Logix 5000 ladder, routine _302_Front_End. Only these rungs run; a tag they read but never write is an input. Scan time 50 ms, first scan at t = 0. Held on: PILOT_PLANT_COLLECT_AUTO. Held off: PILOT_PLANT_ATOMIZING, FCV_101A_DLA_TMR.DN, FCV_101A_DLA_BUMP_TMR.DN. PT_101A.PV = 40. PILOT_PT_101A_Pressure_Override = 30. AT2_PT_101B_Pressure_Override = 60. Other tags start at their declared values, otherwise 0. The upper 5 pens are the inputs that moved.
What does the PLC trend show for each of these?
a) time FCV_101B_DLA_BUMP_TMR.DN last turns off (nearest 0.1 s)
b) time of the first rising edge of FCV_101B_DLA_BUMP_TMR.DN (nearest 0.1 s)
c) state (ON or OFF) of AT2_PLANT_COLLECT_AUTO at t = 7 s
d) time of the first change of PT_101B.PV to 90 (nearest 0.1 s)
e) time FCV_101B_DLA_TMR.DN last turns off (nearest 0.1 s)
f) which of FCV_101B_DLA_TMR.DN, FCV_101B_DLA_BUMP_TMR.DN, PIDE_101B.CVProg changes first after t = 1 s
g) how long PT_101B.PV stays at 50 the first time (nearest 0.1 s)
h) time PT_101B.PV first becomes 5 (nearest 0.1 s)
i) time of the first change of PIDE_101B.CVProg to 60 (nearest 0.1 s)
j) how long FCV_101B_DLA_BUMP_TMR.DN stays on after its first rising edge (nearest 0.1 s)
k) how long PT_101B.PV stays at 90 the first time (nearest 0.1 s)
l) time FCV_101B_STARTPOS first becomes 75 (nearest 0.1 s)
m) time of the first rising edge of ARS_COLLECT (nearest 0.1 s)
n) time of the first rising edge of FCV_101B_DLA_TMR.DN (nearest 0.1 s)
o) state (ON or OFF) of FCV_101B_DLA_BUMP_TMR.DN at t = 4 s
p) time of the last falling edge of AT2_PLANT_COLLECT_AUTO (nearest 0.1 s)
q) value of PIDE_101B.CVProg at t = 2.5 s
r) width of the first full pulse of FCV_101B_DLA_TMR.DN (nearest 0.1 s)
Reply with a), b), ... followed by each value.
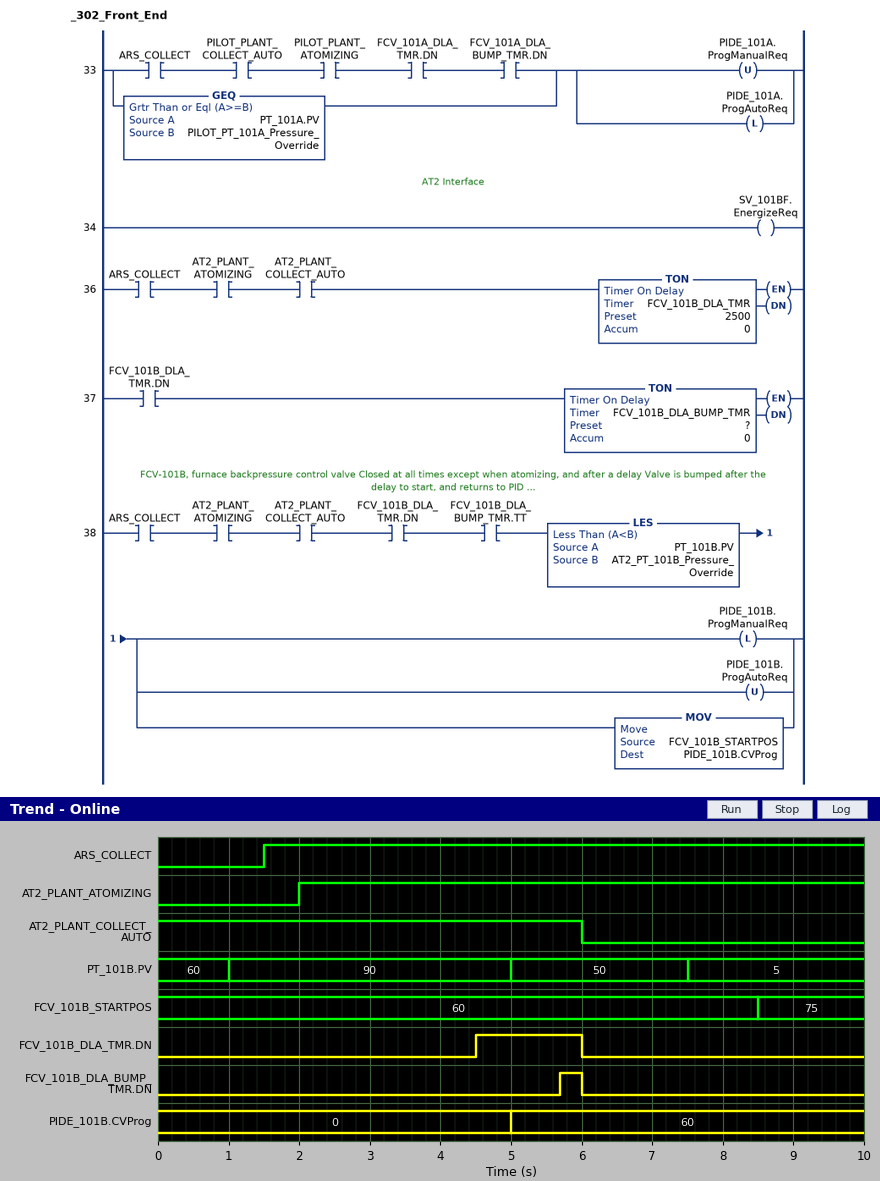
a) 6.0 s
b) 5.7 s
c) OFF
d) 1.0 s
e) 6.0 s
f) FCV_101B_DLA_TMR.DN
g) 2.5 s
h) 7.5 s
i) 5.0 s
j) 0.3 s
k) 4.0 s
l) 8.5 s
m) 1.5 s
n) 4.5 s
o) OFF
p) 6.0 s
q) 0
r) 1.5 s
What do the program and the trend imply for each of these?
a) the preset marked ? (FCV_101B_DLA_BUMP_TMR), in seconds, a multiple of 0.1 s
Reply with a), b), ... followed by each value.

a) 1.2 s
